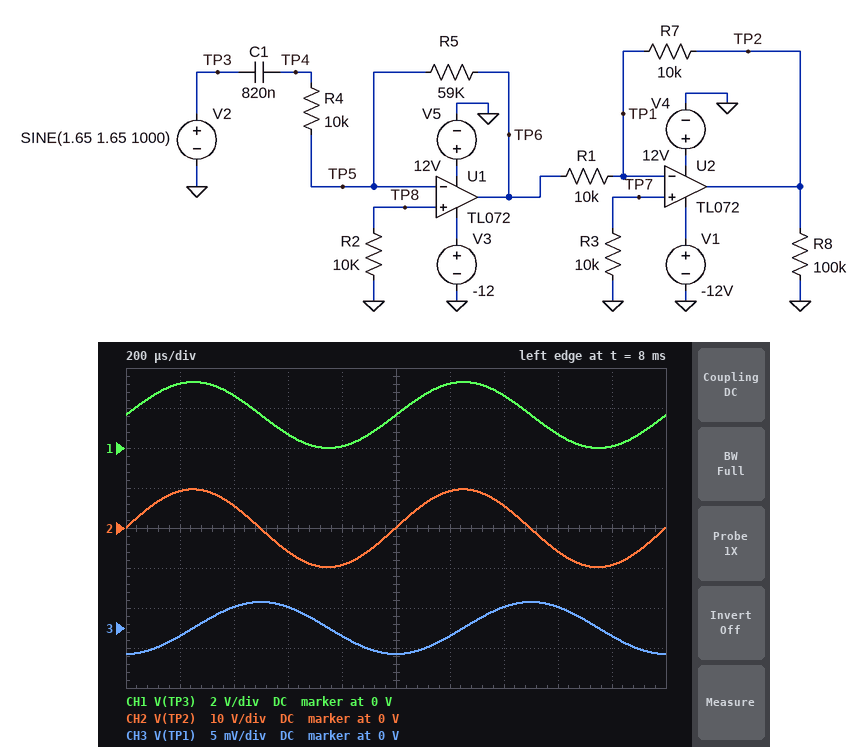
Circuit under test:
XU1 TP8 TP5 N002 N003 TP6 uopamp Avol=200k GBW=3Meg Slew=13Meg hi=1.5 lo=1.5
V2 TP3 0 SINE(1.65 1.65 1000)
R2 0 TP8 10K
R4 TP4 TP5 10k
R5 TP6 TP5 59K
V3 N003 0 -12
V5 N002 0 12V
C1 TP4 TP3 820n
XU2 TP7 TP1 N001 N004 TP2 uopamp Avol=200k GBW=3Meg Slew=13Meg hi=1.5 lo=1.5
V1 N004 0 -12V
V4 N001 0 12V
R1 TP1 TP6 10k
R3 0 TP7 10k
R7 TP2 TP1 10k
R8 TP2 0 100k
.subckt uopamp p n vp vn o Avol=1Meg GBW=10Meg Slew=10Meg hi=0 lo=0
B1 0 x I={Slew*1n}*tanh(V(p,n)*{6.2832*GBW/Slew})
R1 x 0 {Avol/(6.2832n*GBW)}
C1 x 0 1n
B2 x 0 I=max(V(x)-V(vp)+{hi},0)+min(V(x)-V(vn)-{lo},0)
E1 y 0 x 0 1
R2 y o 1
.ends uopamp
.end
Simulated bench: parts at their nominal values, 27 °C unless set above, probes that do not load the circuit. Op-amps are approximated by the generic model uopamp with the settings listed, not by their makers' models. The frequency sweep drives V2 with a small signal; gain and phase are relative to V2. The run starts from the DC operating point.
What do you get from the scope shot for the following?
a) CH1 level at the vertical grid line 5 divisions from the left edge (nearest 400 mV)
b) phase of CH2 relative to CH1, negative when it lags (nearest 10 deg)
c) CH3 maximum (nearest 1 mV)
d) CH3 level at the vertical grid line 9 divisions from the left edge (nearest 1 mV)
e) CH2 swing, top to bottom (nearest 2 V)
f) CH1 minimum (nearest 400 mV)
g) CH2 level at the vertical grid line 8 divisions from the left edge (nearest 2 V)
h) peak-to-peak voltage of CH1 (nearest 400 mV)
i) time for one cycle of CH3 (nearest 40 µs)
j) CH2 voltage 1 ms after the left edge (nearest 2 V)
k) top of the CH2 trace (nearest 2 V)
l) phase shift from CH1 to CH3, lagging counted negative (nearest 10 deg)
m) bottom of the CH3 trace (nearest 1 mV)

1.6 V
0 deg
3 mV
-1 mV
20 V
0 V
-6 V
3.2 V
1.00 ms
0 V
10 V
-90 deg
-3 mV
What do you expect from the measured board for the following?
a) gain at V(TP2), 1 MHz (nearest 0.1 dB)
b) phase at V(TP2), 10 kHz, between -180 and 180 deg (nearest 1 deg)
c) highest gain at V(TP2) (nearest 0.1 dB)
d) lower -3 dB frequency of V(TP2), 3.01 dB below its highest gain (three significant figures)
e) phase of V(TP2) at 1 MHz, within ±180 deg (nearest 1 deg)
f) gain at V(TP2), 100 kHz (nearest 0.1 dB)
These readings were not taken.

5.8 dB
-2 deg
15.4 dB
19.4 Hz
-100 deg
15.2 dB
